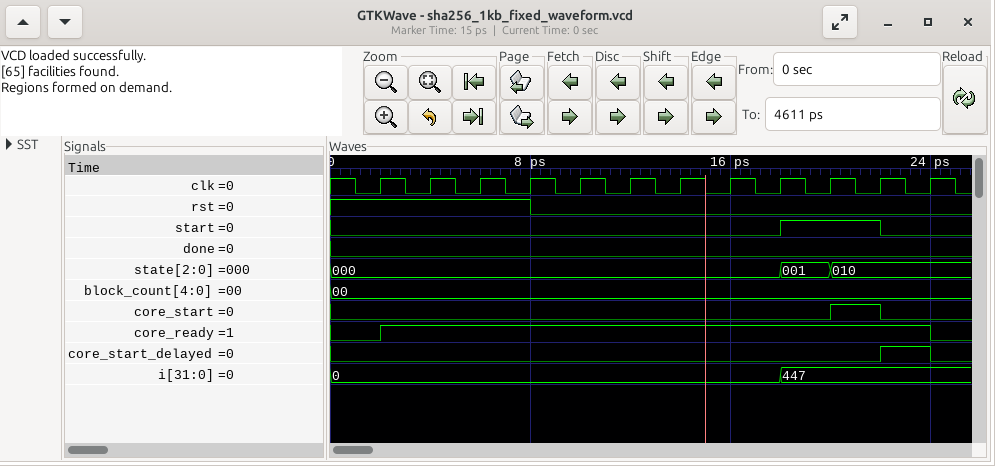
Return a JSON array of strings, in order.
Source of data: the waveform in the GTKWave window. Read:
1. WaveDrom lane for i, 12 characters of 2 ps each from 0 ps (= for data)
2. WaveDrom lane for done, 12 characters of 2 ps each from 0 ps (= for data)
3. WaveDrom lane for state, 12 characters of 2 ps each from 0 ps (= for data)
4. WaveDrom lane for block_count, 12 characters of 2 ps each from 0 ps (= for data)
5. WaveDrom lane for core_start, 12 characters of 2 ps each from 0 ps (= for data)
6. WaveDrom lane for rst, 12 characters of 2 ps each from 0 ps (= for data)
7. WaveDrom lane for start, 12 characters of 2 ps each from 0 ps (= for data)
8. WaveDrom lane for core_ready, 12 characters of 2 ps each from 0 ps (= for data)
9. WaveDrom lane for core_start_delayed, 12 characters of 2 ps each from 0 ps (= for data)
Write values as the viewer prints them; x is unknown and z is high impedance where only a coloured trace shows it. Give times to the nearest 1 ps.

["{name: 'i', wave: '=........=..', data: '0 447'}", "{name: 'done', wave: '0...........'}", "{name: 'state', wave: '=........==.', data: '000 001 010'}", "{name: 'block_count', wave: '=...........', data: '00'}", "{name: 'core_start', wave: '0.........10'}", "{name: 'rst', wave: '1...0.......'}", "{name: 'start', wave: '0........1.0'}", "{name: 'core_ready', wave: '01..........'}", "{name: 'core_start_delayed', wave: '0..........1'}"]
